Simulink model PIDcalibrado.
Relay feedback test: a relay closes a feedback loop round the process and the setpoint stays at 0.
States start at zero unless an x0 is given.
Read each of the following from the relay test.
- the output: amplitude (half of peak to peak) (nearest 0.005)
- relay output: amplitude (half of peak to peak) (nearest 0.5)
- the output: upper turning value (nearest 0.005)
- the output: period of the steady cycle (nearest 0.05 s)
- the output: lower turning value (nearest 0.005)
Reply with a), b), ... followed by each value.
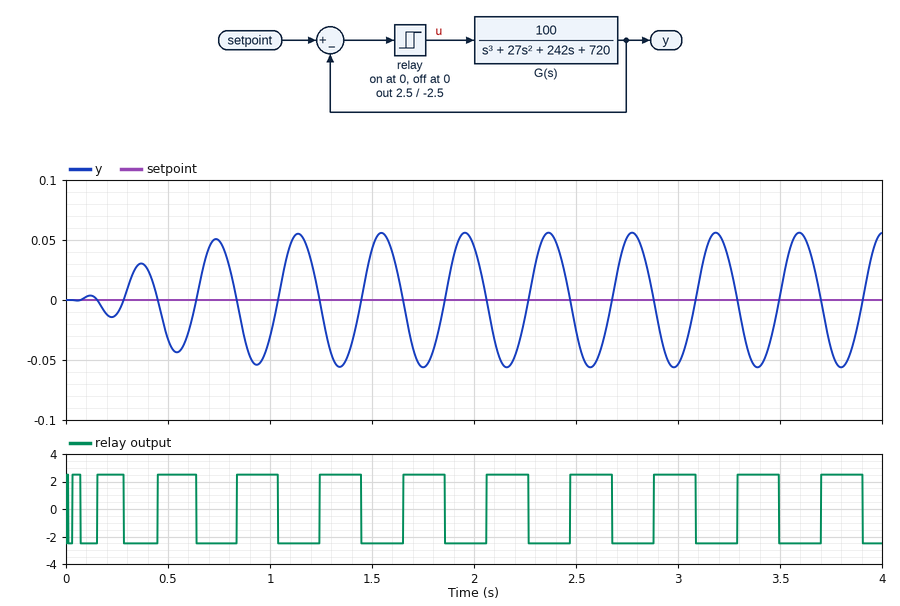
a) 0.055
b) 2.5
c) 0.055
d) 0.40 s
e) -0.055
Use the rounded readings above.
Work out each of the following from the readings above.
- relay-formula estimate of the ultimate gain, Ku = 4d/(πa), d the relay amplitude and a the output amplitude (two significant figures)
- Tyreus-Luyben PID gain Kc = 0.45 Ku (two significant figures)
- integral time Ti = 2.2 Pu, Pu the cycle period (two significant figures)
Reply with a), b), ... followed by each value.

a) 58
b) 26
c) 0.88 s
